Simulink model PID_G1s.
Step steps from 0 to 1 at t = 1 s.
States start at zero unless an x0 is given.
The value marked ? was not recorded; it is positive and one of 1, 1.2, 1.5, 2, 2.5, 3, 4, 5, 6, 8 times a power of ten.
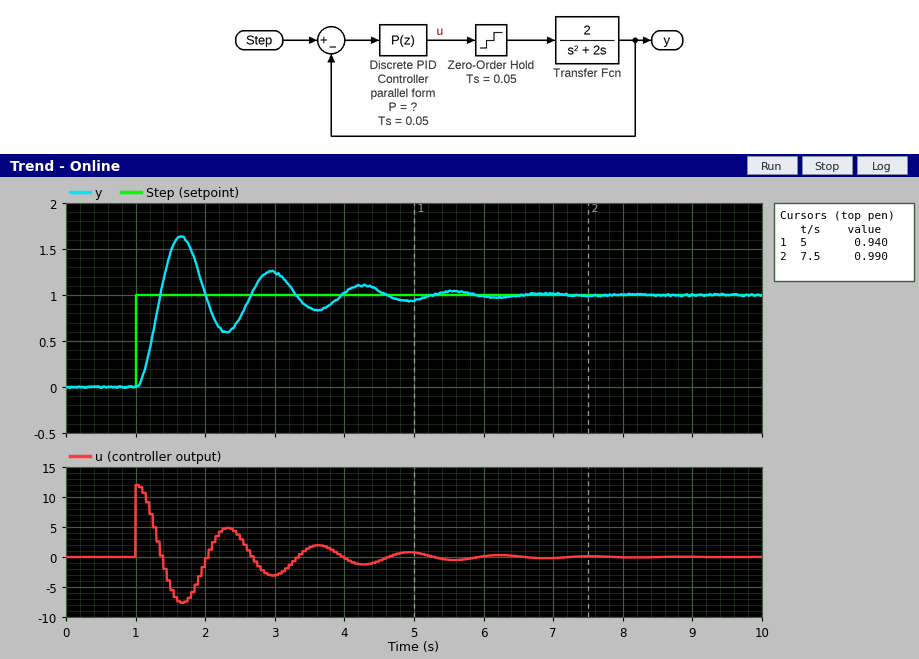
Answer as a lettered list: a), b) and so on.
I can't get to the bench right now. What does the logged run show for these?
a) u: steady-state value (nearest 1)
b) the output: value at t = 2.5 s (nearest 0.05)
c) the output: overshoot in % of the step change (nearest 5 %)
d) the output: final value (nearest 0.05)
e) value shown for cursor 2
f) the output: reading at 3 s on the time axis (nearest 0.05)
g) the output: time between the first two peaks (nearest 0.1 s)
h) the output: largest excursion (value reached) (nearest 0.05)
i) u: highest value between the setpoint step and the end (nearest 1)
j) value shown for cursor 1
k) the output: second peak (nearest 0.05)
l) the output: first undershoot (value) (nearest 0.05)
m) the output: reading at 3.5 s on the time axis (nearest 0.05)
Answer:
a) 0
b) 0.75
c) 65 %
d) 1.00
e) 0.990
f) 1.25
g) 1.3 s
h) 1.65
i) 12
j) 0.940
k) 1.25
l) 0.60
m) 0.85
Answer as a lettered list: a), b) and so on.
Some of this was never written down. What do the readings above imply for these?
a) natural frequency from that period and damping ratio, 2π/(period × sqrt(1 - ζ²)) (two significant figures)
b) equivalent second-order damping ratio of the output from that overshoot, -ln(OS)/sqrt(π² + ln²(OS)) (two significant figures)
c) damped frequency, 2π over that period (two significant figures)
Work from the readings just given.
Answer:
a) 4.9 rad/s
b) 0.14
c) 4.8 rad/s
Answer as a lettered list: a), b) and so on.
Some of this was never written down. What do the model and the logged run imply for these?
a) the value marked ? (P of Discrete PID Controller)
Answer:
a) 12
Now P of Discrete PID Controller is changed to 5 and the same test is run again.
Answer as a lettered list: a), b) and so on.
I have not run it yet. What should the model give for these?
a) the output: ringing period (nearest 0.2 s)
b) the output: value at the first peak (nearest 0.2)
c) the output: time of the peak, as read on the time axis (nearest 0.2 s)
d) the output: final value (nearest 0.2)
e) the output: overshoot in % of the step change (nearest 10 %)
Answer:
a) 2.0 s
b) 1.4
c) 2.0 s
d) 1.0
e) 40 %
